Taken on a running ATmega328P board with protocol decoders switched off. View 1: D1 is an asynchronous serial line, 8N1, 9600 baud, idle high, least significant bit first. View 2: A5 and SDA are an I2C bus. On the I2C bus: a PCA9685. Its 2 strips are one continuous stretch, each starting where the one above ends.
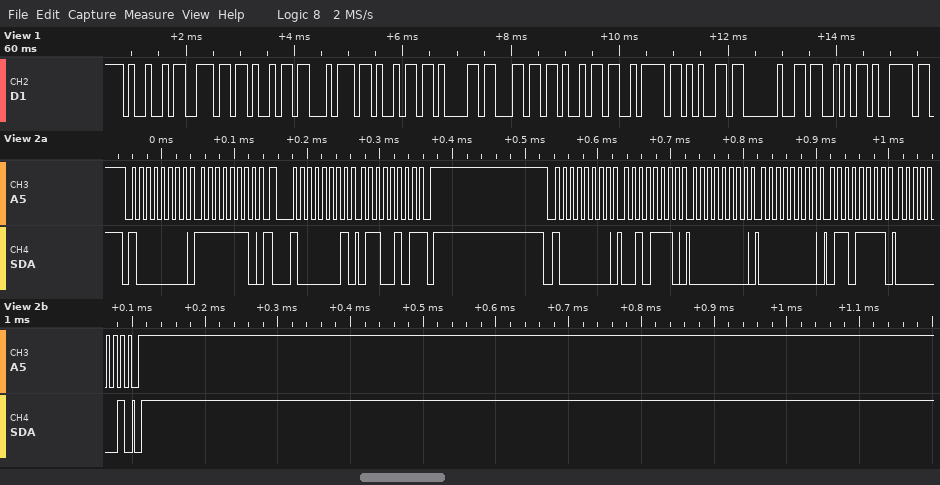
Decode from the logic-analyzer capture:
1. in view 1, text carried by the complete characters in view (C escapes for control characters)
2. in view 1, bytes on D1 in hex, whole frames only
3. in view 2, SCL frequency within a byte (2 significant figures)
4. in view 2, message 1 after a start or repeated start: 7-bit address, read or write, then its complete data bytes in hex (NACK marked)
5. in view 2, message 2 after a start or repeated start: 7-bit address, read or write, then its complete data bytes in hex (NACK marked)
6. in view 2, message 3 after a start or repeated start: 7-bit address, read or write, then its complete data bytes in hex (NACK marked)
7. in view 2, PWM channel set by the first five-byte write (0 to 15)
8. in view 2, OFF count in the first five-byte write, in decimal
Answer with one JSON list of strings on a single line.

["\"Initialize Sy\"", "49 6E 69 74 69 61 6C 69 7A 65 20 53 79", "100 kHz", "0x40 write: FE", "0x40 read: 65 NACK", "0x40 write: 2E 00 00 6F 01", "10", "367"]
